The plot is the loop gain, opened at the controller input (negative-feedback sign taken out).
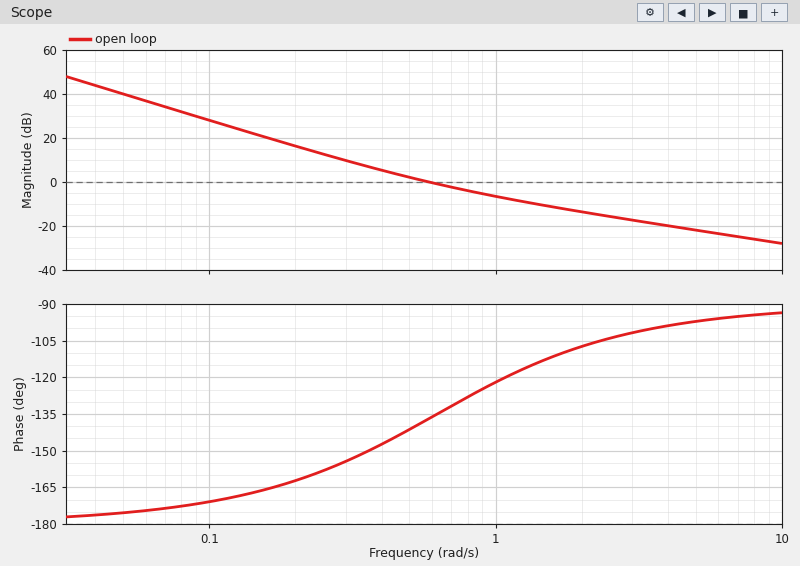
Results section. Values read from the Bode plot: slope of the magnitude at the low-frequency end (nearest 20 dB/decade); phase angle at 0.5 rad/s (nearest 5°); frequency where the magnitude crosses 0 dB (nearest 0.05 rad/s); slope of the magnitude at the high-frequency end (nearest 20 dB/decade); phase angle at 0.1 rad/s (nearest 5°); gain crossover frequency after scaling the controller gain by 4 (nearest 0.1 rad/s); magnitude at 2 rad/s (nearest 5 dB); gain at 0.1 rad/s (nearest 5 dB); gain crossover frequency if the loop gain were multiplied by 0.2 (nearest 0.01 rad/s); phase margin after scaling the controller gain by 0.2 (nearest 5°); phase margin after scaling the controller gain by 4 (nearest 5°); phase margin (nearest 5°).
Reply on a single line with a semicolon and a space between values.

-40 dB/decade; -140°; 0.60 rad/s; -20 dB/decade; -170°; 1.7 rad/s; -15 dB; 30 dB; 0.23 rad/s; 20°; 70°; 45°
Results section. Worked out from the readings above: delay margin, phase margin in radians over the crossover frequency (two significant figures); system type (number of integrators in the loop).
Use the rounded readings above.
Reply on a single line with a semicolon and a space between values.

1.3 s; 2
